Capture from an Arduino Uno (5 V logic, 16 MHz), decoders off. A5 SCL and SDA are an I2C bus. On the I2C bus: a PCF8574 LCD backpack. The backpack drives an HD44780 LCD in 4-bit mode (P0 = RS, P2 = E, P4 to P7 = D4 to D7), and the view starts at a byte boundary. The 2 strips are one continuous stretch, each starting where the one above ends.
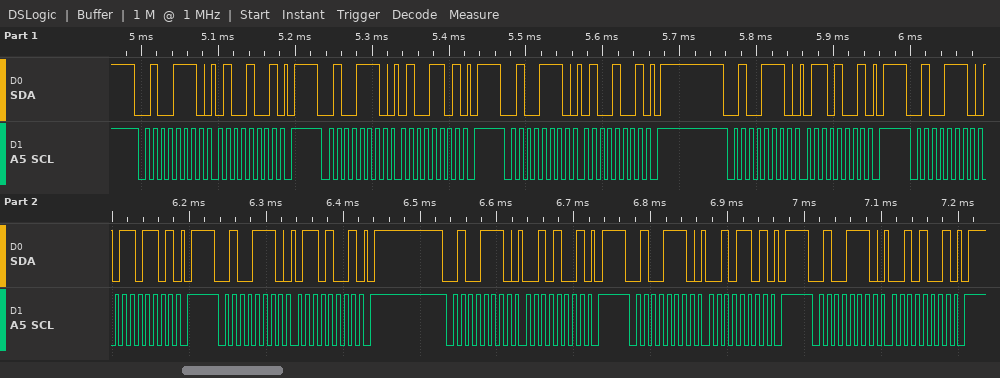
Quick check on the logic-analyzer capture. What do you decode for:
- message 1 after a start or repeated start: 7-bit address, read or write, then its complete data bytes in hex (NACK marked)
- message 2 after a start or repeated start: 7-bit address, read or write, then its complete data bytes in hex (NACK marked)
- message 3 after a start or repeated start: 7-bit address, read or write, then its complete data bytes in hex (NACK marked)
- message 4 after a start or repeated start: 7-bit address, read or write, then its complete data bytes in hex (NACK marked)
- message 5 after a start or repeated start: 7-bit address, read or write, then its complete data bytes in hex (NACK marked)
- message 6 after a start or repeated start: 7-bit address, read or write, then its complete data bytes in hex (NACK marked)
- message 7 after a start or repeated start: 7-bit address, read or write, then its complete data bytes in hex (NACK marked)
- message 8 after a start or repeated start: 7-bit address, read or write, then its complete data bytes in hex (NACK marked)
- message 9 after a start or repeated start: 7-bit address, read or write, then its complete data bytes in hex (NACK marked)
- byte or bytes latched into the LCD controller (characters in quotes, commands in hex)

0x27 write: 49
0x27 write: 4D
0x27 write: 49
0x27 write: 69
0x27 write: 6D
0x27 write: 69
0x27 write: 29
0x27 write: 2D
0x27 write: 29
'F'
